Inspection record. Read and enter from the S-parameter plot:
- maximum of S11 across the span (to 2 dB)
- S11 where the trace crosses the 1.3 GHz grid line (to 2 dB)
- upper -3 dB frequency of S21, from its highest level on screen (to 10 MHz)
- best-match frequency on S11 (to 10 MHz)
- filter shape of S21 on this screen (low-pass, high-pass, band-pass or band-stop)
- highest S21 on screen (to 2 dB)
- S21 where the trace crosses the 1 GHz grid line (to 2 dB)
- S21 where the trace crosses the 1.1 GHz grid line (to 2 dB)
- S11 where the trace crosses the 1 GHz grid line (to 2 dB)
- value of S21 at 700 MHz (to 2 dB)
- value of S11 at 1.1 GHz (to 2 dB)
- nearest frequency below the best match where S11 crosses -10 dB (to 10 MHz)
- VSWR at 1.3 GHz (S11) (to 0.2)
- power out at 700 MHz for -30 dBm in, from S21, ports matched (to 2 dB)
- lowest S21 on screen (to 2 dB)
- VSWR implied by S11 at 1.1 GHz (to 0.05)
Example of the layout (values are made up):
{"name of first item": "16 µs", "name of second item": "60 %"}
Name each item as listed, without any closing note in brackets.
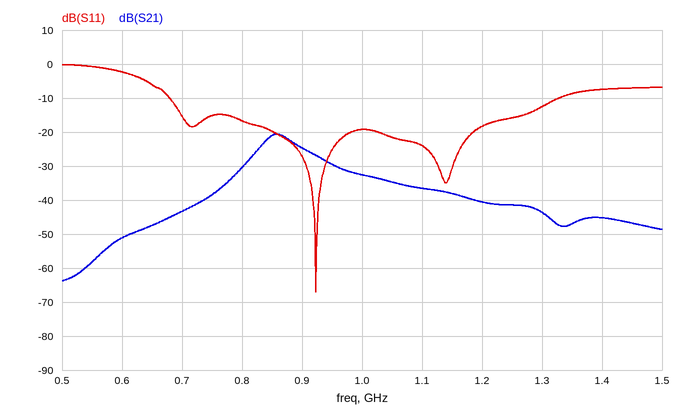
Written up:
{"maximum of S11 across the span": "0 dB", "S11 where the trace crosses the 1.3 GHz grid line": "-12 dB", "upper -3 dB frequency of S21, from its highest level on screen": "890 MHz", "best-match frequency on S11": "920 MHz", "filter shape of S21 on this screen": "band-pass", "highest S21 on screen": "-20 dB", "S21 where the trace crosses the 1 GHz grid line": "-32 dB", "S21 where the trace crosses the 1.1 GHz grid line": "-36 dB", "S11 where the trace crosses the 1 GHz grid line": "-20 dB", "value of S21 at 700 MHz": "-44 dB", "value of S11 at 1.1 GHz": "-24 dB", "nearest frequency below the best match where S11 crosses -10 dB": "680 MHz", "VSWR at 1.3 GHz (S11)": "1.6", "power out at 700 MHz for -30 dBm in, from S21, ports matched": "-74 dBm", "lowest S21 on screen": "-64 dB", "VSWR implied by S11 at 1.1 GHz": "1.15"}
